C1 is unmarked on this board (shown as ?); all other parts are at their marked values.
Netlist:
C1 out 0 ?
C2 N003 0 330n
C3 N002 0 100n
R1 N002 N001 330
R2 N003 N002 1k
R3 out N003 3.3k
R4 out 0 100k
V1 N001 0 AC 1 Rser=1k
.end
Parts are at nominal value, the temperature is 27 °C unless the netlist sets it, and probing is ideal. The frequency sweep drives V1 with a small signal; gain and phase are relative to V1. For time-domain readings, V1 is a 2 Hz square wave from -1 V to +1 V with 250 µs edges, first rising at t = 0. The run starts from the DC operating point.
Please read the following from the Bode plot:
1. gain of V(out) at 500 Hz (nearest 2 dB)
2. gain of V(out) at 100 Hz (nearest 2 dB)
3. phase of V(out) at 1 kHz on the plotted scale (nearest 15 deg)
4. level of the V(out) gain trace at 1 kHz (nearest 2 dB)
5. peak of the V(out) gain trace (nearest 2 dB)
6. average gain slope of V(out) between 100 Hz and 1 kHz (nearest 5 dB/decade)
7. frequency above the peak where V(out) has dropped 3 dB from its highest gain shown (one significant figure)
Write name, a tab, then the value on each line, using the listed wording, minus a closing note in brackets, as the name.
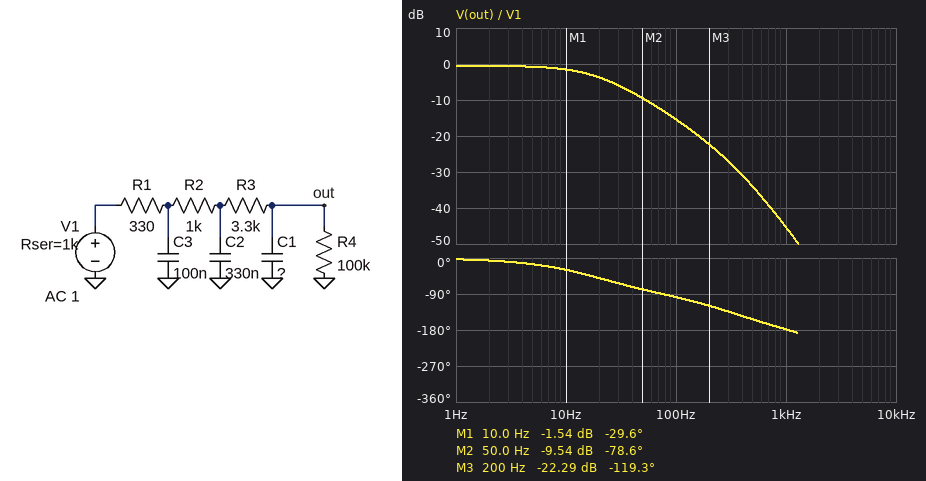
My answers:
gain of V(out) at 500 Hz	-34 dB
gain of V(out) at 100 Hz	-16 dB
phase of V(out) at 1 kHz on the plotted scale	-180 deg
level of the V(out) gain trace at 1 kHz	-46 dB
peak of the V(out) gain trace	0 dB
average gain slope of V(out) between 100 Hz and 1 kHz	-30 dB/decade
frequency above the peak where V(out) has dropped 3 dB from its highest gain shown	20 Hz
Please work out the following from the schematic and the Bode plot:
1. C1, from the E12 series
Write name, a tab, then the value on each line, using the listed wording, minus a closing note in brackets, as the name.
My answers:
C1, from the E12 series	1.5 µF
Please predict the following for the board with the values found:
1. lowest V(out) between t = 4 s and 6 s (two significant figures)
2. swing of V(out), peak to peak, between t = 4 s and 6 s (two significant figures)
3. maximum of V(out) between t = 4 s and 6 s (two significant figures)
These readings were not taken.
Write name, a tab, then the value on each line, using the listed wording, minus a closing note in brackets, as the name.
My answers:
lowest V(out) between t = 4 s and 6 s	-950 mV
swing of V(out), peak to peak, between t = 4 s and 6 s	1.9 V
maximum of V(out) between t = 4 s and 6 s	950 mV
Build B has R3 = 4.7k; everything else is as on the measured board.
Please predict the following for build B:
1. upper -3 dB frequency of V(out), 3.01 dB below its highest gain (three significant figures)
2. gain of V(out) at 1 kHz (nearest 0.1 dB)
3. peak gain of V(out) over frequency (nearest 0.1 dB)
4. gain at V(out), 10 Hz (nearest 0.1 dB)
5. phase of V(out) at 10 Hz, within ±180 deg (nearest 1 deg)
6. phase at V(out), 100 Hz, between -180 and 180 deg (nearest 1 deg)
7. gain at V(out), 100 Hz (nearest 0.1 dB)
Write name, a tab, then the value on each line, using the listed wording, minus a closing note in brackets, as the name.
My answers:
upper -3 dB frequency of V(out), 3.01 dB below its highest gain	15.7 Hz
gain of V(out) at 1 kHz	-48.3 dB
peak gain of V(out) over frequency	-0.6 dB
gain at V(out), 10 Hz	-2.1 dB
phase of V(out) at 10 Hz, within ±180 deg	-35 deg
phase at V(out), 100 Hz, between -180 and 180 deg	-102 deg
gain at V(out), 100 Hz	-17.3 dB
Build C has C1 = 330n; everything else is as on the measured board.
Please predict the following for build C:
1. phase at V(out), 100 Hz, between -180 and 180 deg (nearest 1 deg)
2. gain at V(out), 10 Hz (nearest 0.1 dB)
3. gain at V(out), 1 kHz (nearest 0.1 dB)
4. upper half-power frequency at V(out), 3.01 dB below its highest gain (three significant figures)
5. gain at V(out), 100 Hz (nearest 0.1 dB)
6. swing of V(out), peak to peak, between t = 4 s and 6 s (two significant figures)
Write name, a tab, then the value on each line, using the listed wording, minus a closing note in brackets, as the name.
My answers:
phase at V(out), 100 Hz, between -180 and 180 deg	-70 deg
gain at V(out), 10 Hz	-0.6 dB
gain at V(out), 1 kHz	-32.4 dB
upper half-power frequency at V(out), 3.01 dB below its highest gain	70.4 Hz
gain at V(out), 100 Hz	-5.4 dB
swing of V(out), peak to peak, between t = 4 s and 6 s	1.9 V
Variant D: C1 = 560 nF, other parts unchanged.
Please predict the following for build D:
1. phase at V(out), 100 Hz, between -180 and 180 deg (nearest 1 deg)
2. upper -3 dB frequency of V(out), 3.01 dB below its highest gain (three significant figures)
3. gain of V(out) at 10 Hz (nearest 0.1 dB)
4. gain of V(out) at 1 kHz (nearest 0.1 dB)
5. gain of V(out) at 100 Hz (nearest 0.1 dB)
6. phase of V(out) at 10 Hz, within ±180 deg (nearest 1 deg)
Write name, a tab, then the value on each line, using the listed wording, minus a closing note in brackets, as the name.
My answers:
phase at V(out), 100 Hz, between -180 and 180 deg	-82 deg
upper -3 dB frequency of V(out), 3.01 dB below its highest gain	46.4 Hz
gain of V(out) at 10 Hz	-0.7 dB
gain of V(out) at 1 kHz	-36.9 dB
gain of V(out) at 100 Hz	-8.2 dB
phase of V(out) at 10 Hz, within ±180 deg	-14 deg
